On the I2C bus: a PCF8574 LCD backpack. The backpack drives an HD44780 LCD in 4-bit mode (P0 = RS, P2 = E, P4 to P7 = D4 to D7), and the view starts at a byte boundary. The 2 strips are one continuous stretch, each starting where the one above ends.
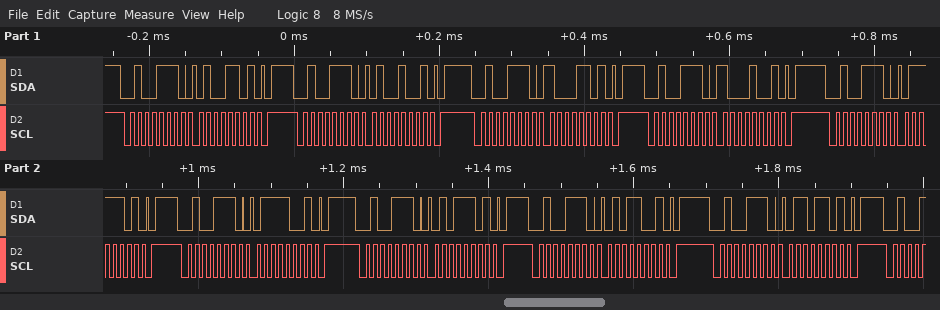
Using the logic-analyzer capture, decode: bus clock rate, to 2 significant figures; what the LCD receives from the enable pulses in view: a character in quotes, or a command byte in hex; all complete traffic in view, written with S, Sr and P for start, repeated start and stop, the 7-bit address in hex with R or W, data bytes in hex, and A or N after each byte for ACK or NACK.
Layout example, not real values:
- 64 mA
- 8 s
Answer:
- 100 kHz
- 'H' 'u'
- S 27W A 4D A P S 27W A 49 A P S 27W A 8D A P S 27W A 89 A P S 27W A 7D A P S 27W A 79 A P S 27W A 5D A P S 27W A 59 A P S 27W A 6D A P
